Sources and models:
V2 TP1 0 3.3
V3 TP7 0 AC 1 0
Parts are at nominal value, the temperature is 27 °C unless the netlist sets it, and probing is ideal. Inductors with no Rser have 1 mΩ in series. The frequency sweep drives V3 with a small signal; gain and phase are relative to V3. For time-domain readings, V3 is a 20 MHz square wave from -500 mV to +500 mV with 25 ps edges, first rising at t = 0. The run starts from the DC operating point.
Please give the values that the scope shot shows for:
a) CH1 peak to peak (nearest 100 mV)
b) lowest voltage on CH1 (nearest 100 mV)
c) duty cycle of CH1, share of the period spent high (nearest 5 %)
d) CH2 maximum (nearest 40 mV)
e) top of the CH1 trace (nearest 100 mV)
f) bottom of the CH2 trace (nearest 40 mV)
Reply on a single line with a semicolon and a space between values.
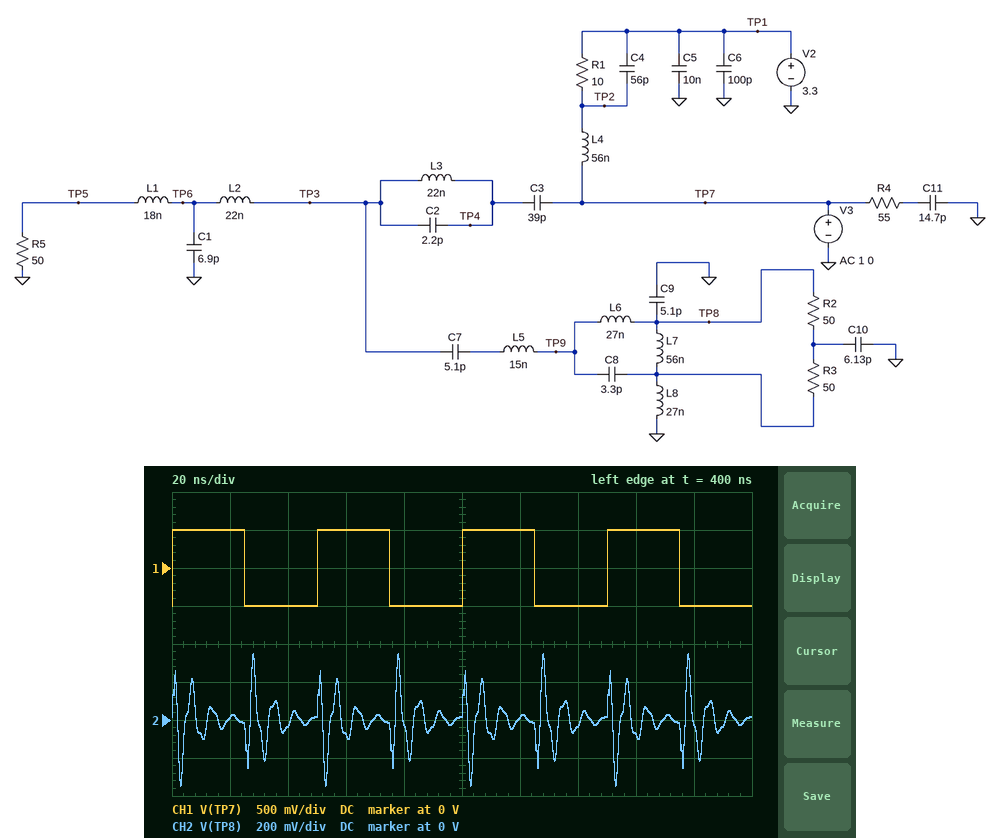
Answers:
1.0 V; -500 mV; 50 %; 360 mV; 500 mV; -360 mV
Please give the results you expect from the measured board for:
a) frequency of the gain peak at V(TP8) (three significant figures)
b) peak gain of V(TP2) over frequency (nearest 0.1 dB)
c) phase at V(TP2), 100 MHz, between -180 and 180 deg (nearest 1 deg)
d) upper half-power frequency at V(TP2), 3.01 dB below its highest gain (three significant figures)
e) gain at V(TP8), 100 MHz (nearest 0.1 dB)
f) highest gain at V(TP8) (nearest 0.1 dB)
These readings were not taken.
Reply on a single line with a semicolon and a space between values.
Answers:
147 MHz; 0 dB; -94 deg; 31.5 MHz; -10.8 dB; 1.6 dB
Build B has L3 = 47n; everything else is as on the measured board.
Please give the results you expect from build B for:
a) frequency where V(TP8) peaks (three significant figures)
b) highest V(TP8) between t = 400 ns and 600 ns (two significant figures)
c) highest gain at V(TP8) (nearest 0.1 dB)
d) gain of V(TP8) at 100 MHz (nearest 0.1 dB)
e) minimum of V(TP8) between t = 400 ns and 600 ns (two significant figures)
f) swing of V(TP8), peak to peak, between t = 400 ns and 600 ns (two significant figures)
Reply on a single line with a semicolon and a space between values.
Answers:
141 MHz; 240 mV; 0.8 dB; -10.0 dB; -240 mV; 480 mV
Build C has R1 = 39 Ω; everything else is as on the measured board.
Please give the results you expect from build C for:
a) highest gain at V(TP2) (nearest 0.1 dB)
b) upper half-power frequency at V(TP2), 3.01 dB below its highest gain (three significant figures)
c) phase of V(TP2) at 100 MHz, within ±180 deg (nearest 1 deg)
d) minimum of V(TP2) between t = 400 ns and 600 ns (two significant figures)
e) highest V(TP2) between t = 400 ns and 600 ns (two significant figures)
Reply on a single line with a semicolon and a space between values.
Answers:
2.6 dB; 107 MHz; -105 deg; -750 mV; 750 mV
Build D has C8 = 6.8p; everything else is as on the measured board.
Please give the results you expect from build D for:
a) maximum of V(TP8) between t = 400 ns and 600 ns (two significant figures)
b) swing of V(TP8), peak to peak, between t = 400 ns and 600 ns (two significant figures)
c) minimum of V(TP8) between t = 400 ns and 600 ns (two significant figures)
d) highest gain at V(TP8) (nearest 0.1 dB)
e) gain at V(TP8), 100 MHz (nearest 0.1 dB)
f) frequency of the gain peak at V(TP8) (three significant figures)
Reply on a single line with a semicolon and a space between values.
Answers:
240 mV; 490 mV; -240 mV; 0.1 dB; -9.7 dB; 137 MHz
